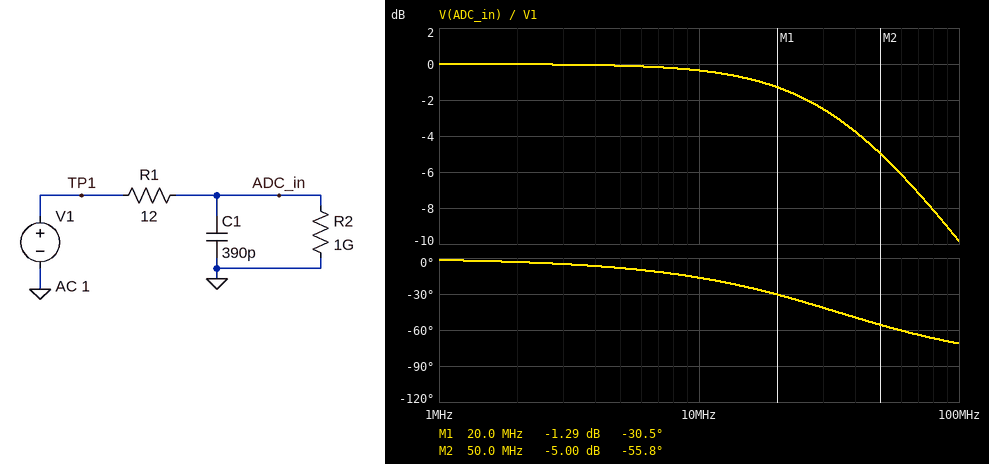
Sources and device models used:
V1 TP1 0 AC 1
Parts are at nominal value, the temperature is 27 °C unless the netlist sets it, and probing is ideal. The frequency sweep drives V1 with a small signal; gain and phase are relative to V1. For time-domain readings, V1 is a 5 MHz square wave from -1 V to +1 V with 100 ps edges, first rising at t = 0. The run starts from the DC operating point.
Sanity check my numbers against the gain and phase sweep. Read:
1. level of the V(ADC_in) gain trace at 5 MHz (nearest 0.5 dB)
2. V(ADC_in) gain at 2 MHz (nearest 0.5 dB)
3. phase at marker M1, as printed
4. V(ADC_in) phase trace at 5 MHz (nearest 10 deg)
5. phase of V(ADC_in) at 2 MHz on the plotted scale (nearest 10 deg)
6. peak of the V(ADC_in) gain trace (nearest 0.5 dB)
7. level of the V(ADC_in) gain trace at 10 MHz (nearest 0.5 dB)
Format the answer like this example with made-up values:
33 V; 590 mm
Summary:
0 dB; 0 dB; -30.5 deg; -10 deg; 0 deg; 0 dB; -0.5 dB
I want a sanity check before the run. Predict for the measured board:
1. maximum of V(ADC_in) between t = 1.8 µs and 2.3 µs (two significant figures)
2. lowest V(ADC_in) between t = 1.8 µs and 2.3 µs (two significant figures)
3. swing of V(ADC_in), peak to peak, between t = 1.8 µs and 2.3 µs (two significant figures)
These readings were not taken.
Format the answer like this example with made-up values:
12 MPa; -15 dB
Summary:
1.0 V; -1.0 V; 2.0 V
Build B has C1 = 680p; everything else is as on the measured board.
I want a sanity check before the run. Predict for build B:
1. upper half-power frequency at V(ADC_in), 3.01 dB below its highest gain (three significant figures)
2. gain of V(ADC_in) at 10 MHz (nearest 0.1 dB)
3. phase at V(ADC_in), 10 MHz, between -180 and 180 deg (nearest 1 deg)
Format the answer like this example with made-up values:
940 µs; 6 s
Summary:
19.5 MHz; -1.0 dB; -27 deg
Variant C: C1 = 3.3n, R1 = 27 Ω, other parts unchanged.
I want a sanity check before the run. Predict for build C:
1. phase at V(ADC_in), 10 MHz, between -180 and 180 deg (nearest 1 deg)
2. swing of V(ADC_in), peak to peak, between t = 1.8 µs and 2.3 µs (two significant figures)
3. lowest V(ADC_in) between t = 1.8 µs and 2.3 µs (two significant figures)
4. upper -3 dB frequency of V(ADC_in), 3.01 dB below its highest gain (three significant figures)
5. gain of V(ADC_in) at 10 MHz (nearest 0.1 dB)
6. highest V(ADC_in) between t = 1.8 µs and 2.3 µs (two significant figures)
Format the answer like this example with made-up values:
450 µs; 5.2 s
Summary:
-80 deg; 1.0 V; -510 mV; 1.79 MHz; -15.1 dB; 510 mV
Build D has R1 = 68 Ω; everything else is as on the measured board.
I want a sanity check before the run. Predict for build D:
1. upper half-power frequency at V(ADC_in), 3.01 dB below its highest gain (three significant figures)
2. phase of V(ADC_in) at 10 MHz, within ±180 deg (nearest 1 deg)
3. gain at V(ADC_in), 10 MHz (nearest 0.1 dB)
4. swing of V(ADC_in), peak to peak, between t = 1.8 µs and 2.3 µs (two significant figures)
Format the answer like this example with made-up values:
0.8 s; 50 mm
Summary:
6.00 MHz; -59 deg; -5.8 dB; 1.9 V
